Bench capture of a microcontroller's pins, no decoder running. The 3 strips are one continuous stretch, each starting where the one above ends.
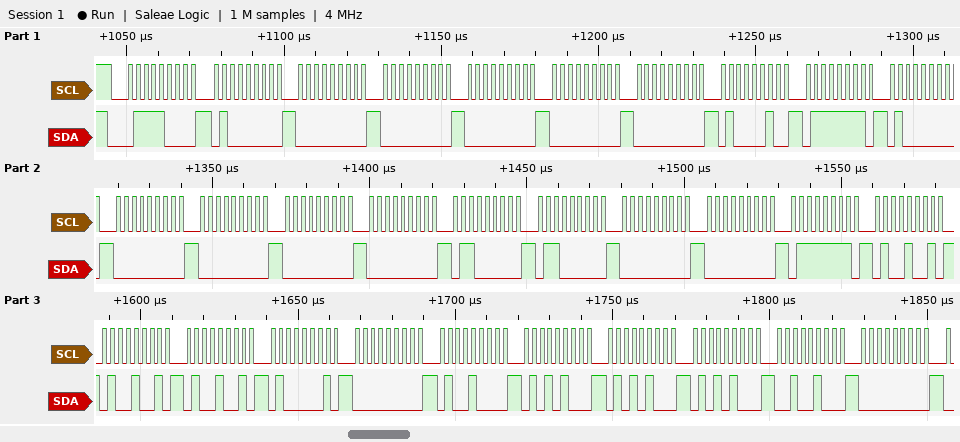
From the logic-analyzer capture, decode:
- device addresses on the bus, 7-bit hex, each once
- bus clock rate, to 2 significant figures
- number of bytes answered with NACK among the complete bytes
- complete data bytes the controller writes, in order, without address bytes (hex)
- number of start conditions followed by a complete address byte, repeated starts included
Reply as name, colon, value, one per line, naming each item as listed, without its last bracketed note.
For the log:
device addresses on the bus, 7-bit hex, each once: 0x3C
bus clock rate, to 2 significant figures: 400 kHz
number of bytes answered with NACK among the complete bytes: 0
complete data bytes the controller writes, in order, without address bytes: 40 00 00 00 00 00 42 7F 40 00 00 00 00 60 60 00 00 7F 49 49 49 41 00 48 54 54 54 24 00
number of start conditions followed by a complete address byte, repeated starts included: 1
